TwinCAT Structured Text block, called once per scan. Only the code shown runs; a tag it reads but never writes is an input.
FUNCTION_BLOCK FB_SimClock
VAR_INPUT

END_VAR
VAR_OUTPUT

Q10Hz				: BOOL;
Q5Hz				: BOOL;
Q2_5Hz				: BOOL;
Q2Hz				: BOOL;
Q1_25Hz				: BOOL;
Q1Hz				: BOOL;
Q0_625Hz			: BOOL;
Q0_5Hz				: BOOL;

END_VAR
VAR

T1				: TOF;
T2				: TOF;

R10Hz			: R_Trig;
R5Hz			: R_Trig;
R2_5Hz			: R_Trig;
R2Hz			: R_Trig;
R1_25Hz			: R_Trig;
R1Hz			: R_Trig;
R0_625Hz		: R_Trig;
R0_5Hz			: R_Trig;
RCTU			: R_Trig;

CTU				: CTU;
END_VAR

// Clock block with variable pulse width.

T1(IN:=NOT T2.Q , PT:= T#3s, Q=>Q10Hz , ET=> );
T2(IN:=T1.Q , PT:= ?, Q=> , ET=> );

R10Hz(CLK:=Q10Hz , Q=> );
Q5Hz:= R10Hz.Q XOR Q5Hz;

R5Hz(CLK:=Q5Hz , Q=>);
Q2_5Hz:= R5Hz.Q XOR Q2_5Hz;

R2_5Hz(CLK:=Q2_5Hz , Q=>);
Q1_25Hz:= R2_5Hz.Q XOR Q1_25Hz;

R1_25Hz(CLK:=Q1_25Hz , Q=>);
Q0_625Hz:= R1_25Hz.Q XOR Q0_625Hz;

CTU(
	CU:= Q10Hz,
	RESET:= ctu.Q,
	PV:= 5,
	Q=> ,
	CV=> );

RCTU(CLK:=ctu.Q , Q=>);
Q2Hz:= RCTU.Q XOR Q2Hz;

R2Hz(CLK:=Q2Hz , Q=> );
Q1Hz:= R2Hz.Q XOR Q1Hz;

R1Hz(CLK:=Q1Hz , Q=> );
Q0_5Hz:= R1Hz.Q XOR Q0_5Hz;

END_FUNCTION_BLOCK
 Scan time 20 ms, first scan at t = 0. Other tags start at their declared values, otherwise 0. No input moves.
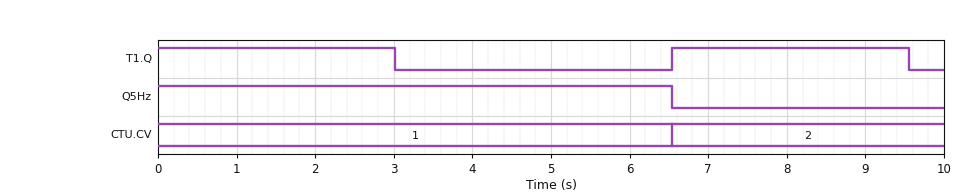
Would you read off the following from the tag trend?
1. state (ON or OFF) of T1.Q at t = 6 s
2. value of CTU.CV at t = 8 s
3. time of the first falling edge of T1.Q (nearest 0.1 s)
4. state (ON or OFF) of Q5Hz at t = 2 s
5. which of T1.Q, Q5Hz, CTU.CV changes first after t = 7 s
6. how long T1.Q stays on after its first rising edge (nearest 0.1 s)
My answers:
OFF
2
3.0 s
ON
T1.Q
3.0 s
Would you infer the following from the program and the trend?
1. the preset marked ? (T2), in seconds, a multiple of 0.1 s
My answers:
3.5 s
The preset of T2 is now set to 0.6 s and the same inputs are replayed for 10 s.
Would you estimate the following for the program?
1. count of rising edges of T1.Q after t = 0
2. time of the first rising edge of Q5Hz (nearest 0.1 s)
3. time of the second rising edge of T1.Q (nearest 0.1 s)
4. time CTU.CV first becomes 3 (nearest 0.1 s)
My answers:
2
7.3 s
7.3 s
7.3 s
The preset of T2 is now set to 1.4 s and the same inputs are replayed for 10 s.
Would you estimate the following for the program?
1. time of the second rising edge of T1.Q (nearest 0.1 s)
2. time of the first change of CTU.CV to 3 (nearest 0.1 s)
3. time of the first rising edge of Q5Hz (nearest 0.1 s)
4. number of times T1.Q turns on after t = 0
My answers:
8.9 s
8.9 s
8.9 s
2
